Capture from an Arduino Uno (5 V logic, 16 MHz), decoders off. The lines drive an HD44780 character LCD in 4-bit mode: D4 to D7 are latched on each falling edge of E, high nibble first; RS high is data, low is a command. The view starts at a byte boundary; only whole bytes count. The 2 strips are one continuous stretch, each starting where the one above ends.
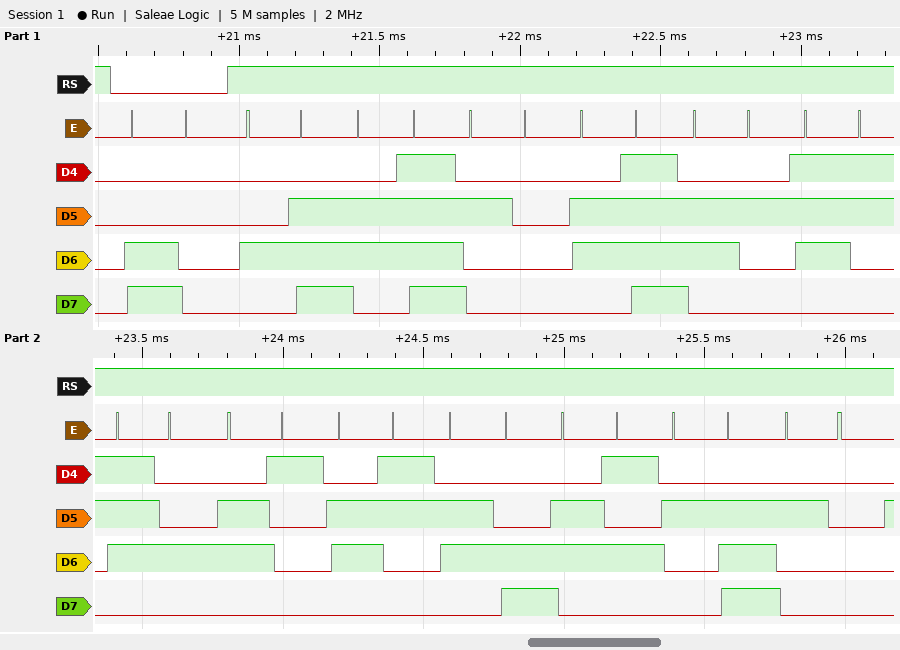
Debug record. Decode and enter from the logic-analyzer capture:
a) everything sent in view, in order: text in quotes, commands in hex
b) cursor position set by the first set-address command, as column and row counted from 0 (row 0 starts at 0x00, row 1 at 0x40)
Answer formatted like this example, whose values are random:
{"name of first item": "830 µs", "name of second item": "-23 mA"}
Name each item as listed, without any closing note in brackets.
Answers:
{"everything sent in view, in order: text in quotes, commands in hex": "0xC0 \"No obstacle. \"", "cursor position set by the first set-address command, as column and row counted from 0": "column 0, row 1"}
